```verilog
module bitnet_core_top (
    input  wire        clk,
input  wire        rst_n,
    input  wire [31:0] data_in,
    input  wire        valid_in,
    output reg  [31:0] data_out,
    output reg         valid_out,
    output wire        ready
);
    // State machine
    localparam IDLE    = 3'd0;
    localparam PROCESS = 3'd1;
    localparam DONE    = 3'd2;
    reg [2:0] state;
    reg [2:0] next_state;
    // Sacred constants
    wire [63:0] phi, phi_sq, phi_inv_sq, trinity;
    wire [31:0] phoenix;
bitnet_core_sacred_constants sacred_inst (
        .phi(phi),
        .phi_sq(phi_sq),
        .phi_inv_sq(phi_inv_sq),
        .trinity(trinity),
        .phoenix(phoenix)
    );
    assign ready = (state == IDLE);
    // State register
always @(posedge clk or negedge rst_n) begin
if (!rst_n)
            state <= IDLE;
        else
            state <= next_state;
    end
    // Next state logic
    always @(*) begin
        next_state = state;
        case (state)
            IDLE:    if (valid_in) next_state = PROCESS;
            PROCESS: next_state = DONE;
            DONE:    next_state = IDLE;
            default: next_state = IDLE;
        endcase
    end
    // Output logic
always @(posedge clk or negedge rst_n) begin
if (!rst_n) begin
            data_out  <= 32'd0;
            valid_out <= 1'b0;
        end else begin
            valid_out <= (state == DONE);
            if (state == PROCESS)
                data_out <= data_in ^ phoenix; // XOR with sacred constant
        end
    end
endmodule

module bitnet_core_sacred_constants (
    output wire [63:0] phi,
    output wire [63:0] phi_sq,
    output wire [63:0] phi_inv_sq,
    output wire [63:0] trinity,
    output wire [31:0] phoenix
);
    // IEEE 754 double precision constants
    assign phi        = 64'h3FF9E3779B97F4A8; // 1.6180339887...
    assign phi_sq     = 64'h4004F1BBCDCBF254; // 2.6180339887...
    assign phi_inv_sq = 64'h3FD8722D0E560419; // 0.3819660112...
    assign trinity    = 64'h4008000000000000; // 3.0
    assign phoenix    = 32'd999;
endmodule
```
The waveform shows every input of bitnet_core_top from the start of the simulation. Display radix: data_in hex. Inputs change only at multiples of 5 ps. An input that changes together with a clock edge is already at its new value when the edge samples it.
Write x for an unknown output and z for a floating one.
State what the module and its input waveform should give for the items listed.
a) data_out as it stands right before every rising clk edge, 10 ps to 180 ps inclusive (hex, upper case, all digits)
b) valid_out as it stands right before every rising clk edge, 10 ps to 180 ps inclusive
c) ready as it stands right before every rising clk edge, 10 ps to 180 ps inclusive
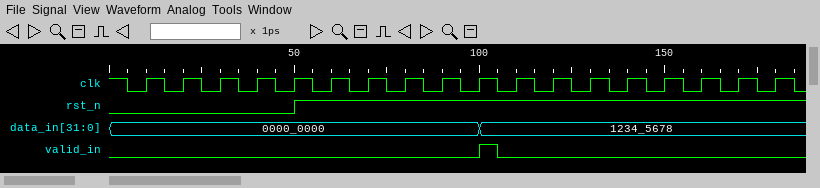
00000000, 00000000, 00000000, 00000000, 00000000, 00000000, 00000000, 00000000, 00000000, 00000000, 00000000, 1234559F, 1234559F, 1234559F, 1234559F, 1234559F, 1234559F, 1234559F
0 0 0 0 0 0 0 0 0 0 0 0 1 0 0 0 0 0
1 1 1 1 1 1 1 1 1 1 0 0 1 1 1 1 1 1
